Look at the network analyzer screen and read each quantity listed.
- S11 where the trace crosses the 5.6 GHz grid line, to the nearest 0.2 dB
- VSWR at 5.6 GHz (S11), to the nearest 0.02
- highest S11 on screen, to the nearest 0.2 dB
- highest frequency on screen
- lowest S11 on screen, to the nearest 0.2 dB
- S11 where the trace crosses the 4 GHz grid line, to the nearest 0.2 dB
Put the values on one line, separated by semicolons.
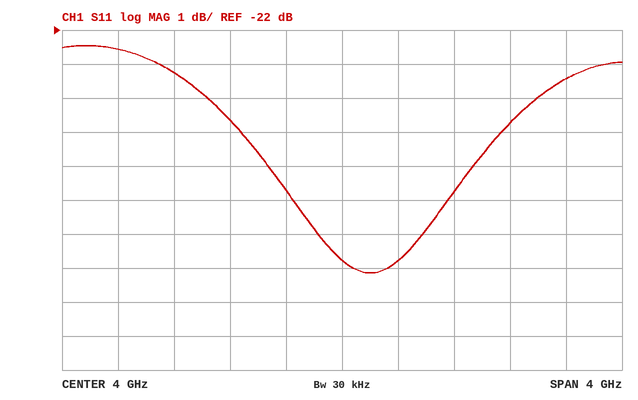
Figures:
-23.4 dB; 1.14; -22.4 dB; 6 GHz; -29.2 dB; -28.8 dB
